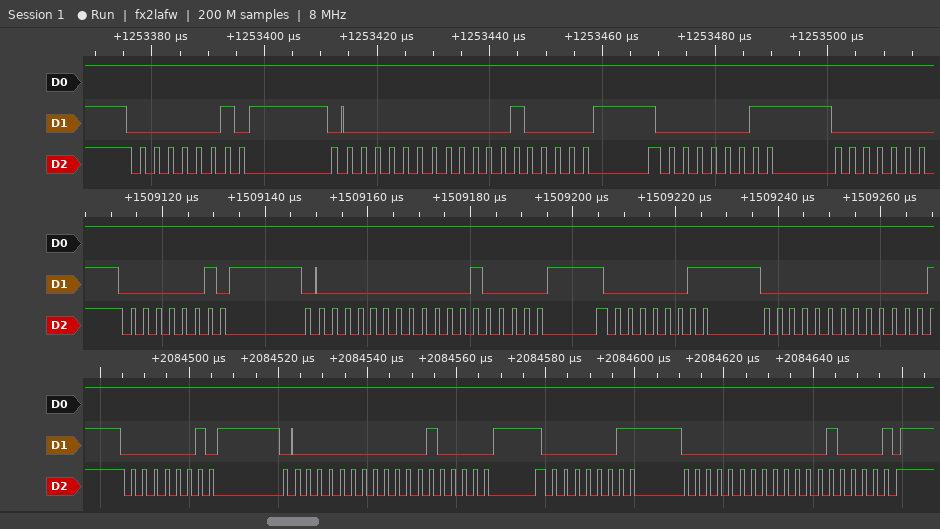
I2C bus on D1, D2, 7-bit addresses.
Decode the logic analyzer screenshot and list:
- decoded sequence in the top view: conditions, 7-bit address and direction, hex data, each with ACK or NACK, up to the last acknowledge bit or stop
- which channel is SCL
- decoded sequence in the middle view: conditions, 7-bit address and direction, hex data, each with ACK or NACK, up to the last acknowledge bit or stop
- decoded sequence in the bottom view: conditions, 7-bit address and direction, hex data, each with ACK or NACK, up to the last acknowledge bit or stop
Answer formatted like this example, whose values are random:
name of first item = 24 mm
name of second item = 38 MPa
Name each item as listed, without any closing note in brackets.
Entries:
decoded sequence in the top view: conditions, 7-bit address and direction, hex data, each with ACK or NACK, up to the last acknowledge bit or stop = start, address 01 write ACK, 00 ACK, 10 ACK, repeated start, address 01 read ACK
which channel is SCL = D2
decoded sequence in the middle view: conditions, 7-bit address and direction, hex data, each with ACK or NACK, up to the last acknowledge bit or stop = start, address 01 write ACK, 00 ACK, 10 ACK, repeated start, address 01 read ACK, 00 ACK
decoded sequence in the bottom view: conditions, 7-bit address and direction, hex data, each with ACK or NACK, up to the last acknowledge bit or stop = start, address 01 write ACK, 00 ACK, 10 ACK, repeated start, address 01 read ACK, 00 ACK, 10 NACK, stop
